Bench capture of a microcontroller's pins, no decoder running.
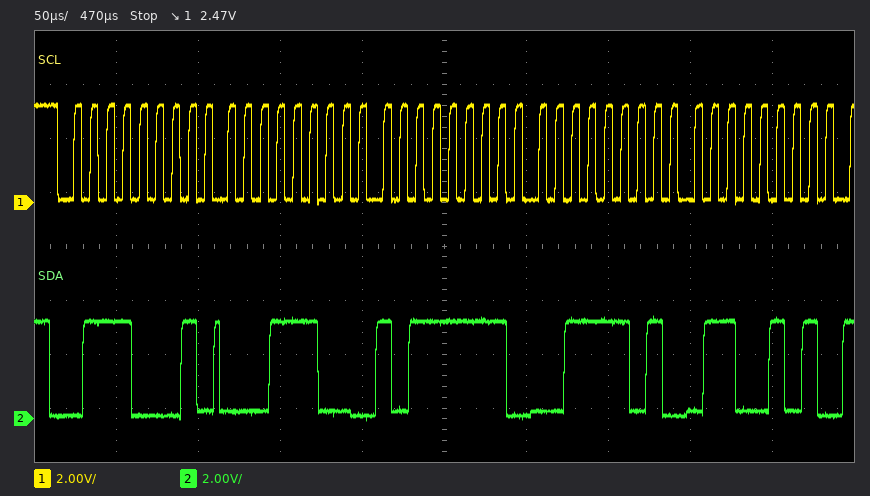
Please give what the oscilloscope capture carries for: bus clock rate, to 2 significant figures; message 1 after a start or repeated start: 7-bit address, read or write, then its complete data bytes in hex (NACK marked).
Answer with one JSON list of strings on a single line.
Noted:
["100 kHz", "0x38 read: 1C BF 3D 65"]
